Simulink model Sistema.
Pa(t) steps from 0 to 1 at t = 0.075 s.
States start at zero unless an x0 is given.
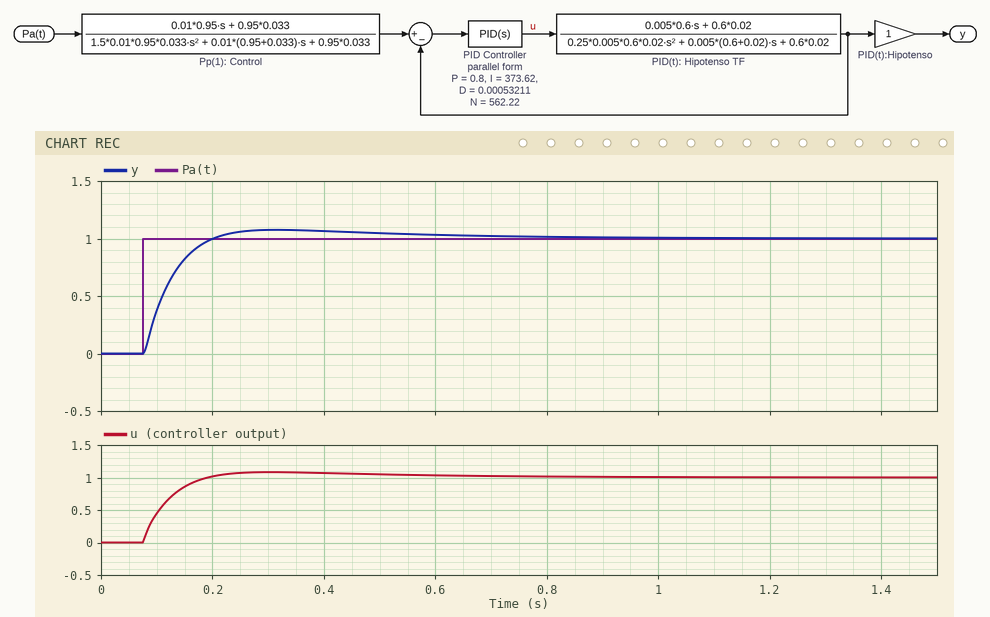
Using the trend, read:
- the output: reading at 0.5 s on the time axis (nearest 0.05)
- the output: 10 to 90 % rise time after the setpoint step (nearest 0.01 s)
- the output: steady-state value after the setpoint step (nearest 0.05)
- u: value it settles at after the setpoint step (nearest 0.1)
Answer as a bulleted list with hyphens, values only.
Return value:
- 1.05
- 0.08 s
- 1.00
- 1.0
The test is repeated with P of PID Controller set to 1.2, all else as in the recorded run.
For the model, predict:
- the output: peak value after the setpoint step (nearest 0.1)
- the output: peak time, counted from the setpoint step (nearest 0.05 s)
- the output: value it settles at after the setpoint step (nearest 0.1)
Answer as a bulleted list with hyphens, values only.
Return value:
- 1.1
- 0.25 s
- 1.0
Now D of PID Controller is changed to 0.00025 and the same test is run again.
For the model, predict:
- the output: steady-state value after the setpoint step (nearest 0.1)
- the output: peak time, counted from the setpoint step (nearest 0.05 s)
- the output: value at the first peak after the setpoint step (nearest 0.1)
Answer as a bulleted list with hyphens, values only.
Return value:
- 1.0
- 0.25 s
- 1.1
